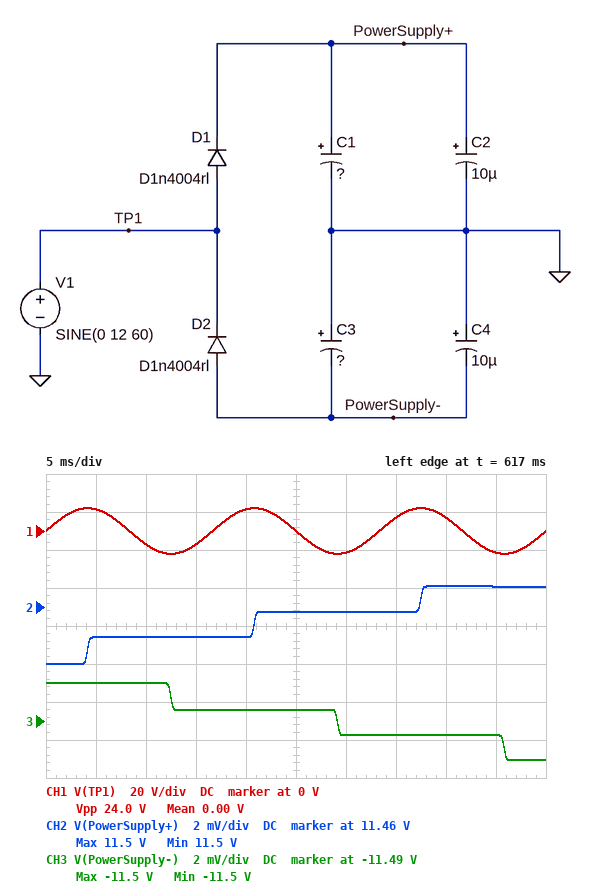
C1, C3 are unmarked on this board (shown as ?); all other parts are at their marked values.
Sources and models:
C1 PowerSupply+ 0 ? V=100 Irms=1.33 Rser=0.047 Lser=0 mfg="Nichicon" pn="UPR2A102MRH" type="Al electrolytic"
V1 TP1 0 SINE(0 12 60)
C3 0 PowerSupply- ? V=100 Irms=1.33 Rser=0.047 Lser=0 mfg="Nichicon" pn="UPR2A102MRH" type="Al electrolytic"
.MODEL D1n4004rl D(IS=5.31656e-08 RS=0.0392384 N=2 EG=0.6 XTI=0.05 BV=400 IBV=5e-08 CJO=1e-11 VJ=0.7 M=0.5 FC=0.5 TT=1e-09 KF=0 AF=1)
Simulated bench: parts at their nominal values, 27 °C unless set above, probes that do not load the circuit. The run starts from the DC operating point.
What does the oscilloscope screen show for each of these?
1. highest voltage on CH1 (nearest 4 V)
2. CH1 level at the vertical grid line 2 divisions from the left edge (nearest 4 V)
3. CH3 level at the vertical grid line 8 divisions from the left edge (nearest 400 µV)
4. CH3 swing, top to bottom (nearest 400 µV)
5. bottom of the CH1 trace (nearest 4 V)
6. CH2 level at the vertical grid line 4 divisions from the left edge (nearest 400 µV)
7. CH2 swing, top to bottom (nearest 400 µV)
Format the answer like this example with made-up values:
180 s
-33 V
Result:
12 V
-8 V
-11.4888 V
4.0 mV
-12 V
11.4604 V
4.0 mV
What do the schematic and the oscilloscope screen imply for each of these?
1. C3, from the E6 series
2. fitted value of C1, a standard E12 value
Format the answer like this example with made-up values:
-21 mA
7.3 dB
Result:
330 µF
560 µF
